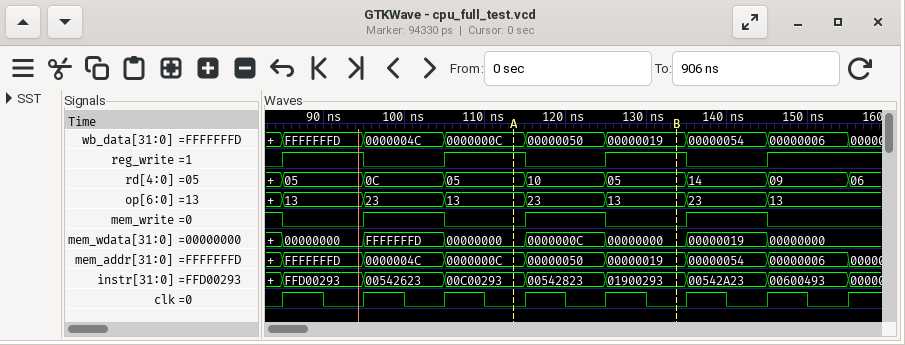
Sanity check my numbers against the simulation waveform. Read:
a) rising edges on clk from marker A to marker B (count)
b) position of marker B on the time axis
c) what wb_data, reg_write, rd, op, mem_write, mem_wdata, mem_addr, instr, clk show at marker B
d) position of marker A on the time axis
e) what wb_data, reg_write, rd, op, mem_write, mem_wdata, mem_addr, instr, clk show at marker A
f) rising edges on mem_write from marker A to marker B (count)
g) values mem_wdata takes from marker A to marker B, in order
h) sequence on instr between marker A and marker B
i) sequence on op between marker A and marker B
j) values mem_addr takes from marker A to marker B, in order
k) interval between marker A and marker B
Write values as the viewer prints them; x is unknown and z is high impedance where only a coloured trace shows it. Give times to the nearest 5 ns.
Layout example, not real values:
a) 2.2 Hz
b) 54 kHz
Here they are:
a) 2
b) 135 ns
c) wb_data=00000019, reg_write=1, rd=05, op=13, mem_write=0, mem_wdata=00000000, mem_addr=00000019, instr=01900293, clk=0
d) 115 ns
e) wb_data=0000000C, reg_write=1, rd=05, op=13, mem_write=0, mem_wdata=00000000, mem_addr=0000000C, instr=00C00293, clk=0
f) 1
g) 00000000, 0000000C, 00000000
h) 00C00293, 00542823, 01900293
i) 13, 23, 13
j) 0000000C, 00000050, 00000019
k) 20 ns
